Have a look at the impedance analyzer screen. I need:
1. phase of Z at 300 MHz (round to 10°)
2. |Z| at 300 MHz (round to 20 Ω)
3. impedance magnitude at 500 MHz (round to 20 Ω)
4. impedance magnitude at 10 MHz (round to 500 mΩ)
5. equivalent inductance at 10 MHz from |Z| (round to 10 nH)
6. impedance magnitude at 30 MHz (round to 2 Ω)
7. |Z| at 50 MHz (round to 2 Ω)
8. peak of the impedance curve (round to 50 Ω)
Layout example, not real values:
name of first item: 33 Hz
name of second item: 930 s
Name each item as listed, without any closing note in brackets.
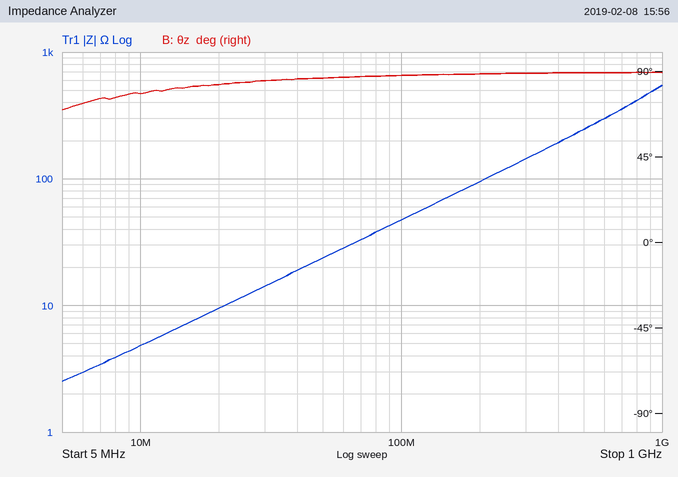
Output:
phase of Z at 300 MHz: 90°
|Z| at 300 MHz: 140 Ω
impedance magnitude at 500 MHz: 240 Ω
impedance magnitude at 10 MHz: 5.0 Ω
equivalent inductance at 10 MHz from |Z|: 80 nH
impedance magnitude at 30 MHz: 14 Ω
|Z| at 50 MHz: 24 Ω
peak of the impedance curve: 550 Ω
